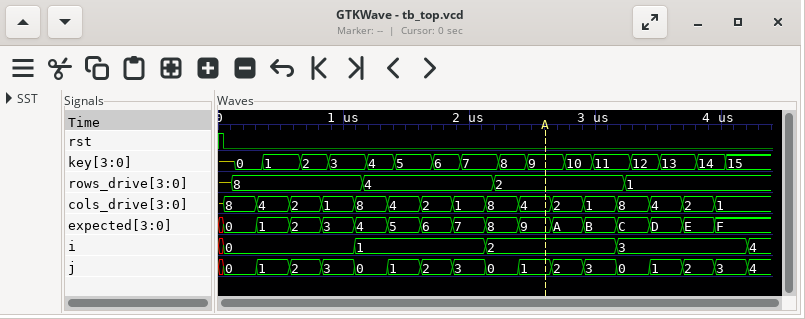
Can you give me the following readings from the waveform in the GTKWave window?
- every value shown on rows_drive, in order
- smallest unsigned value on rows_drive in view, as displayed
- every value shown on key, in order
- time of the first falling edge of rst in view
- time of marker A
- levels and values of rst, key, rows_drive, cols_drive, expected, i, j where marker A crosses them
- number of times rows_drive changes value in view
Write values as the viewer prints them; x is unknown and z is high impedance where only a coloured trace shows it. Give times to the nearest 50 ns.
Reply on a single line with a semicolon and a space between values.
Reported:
z, 8, 4, 2, 1; 1; z, 0, 1, 2, 3, 4, 5, 6, 7, 8, 9, 10, 11, 12, 13, 14, 15; 50 ns; 2600 ns; rst=0, key=9, rows_drive=2, cols_drive=4, expected=9, i=2, j=1; 4
